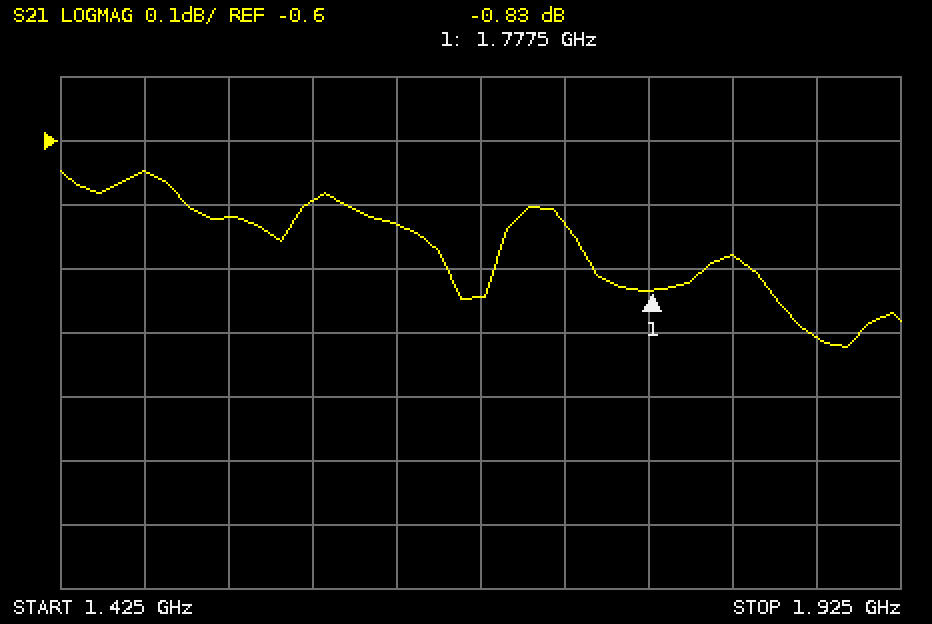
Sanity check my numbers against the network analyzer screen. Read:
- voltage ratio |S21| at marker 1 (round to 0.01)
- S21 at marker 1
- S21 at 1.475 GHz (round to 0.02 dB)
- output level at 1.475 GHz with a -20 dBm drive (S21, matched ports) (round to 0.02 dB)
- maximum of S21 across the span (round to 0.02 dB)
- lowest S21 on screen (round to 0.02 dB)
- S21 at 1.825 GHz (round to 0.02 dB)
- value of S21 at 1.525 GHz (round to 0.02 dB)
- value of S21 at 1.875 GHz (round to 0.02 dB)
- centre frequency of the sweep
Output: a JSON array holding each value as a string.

["0.91", "-0.83 dB", "-0.64 dB", "-20.64 dBm", "-0.64 dB", "-0.92 dB", "-0.78 dB", "-0.72 dB", "-0.90 dB", "1.675 GHz"]
